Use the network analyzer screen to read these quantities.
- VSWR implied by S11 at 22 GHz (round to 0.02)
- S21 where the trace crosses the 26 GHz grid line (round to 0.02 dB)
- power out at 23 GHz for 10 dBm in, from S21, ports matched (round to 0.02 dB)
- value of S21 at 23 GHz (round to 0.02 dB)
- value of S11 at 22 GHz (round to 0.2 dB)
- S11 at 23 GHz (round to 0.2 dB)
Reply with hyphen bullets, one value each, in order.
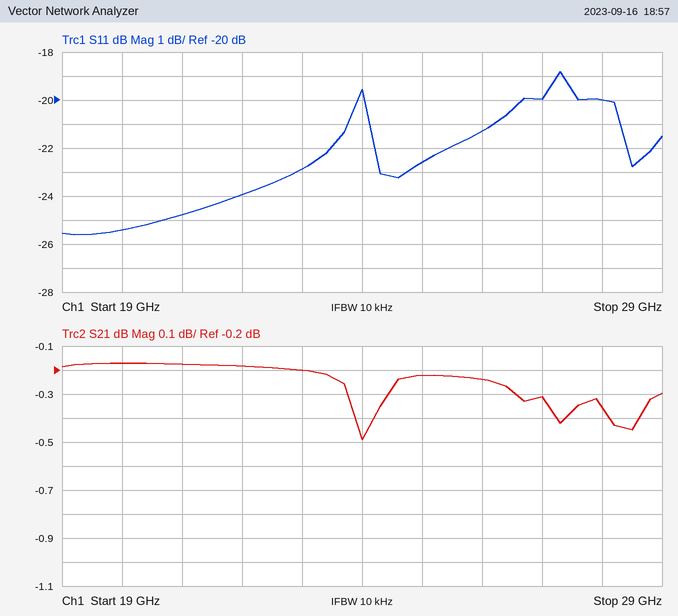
- 1.14
- -0.24 dB
- 9.80 dBm
- -0.20 dB
- -24.0 dB
- -22.8 dB
